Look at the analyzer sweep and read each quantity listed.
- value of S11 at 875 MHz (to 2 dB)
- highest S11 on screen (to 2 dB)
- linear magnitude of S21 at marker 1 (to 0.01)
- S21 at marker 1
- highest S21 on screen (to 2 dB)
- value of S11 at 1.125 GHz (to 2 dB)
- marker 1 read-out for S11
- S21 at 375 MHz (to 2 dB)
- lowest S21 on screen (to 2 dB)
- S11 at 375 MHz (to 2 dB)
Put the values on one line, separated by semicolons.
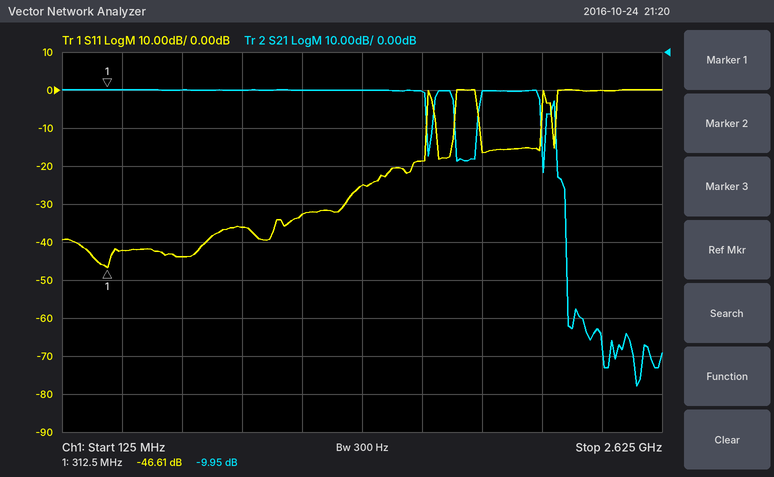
-36 dB; 0 dB; 0.32; -9.95 dB; -10 dB; -32 dB; -46.61 dB; -10 dB; -88 dB; -42 dB
